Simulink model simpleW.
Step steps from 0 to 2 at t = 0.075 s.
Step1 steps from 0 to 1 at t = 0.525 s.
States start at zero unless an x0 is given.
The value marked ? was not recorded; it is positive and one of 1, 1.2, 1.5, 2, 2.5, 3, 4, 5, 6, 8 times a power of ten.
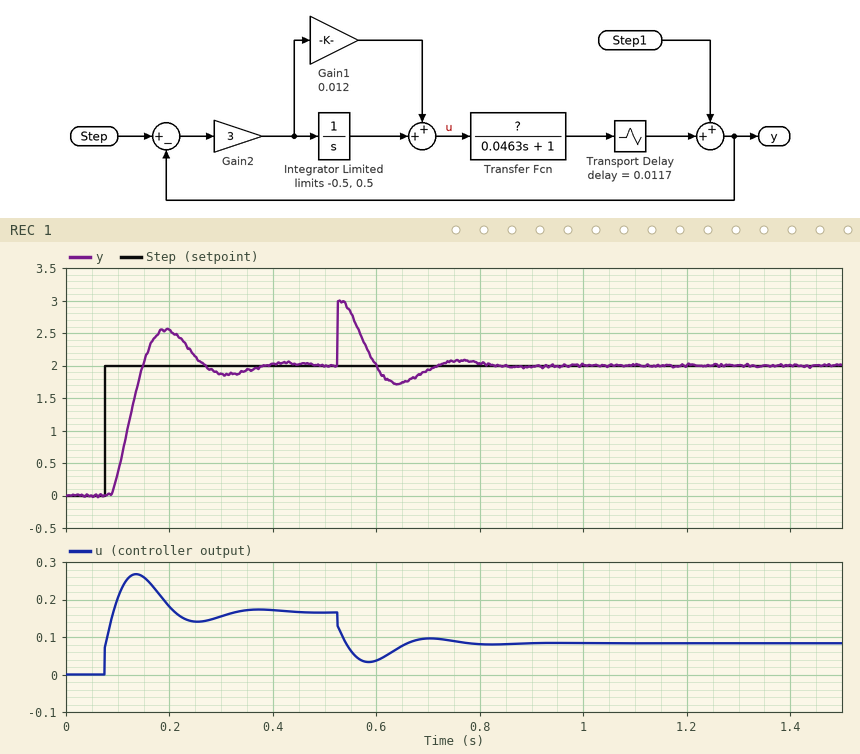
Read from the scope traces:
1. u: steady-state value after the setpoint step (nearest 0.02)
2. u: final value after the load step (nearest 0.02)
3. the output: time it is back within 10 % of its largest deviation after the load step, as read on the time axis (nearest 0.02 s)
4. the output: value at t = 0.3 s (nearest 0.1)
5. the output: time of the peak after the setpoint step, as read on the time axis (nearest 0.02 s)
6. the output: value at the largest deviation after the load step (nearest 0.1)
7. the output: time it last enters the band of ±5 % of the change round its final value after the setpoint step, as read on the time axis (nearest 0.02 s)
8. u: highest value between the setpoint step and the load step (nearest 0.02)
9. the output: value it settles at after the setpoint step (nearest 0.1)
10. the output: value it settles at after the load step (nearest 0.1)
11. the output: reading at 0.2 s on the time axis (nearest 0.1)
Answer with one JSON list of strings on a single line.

["0.16", "0.08", "0.70 s", "1.9", "0.20 s", "3.0", "0.34 s", "0.26", "2.0", "2.0", "2.5"]
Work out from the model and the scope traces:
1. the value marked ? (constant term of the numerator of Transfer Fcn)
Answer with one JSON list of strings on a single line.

["12"]
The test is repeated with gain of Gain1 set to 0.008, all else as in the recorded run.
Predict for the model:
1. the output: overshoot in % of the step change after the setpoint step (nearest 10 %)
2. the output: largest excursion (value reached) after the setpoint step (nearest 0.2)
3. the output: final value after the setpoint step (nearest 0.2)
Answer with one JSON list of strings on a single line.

["30 %", "2.6", "2.0"]
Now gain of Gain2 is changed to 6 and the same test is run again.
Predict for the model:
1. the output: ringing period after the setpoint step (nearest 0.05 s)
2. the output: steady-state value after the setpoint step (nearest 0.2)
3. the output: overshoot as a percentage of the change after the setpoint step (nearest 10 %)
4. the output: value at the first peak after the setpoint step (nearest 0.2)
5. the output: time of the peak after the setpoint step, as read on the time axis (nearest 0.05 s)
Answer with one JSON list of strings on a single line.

["0.15 s", "2.0", "50 %", "3.0", "0.15 s"]
